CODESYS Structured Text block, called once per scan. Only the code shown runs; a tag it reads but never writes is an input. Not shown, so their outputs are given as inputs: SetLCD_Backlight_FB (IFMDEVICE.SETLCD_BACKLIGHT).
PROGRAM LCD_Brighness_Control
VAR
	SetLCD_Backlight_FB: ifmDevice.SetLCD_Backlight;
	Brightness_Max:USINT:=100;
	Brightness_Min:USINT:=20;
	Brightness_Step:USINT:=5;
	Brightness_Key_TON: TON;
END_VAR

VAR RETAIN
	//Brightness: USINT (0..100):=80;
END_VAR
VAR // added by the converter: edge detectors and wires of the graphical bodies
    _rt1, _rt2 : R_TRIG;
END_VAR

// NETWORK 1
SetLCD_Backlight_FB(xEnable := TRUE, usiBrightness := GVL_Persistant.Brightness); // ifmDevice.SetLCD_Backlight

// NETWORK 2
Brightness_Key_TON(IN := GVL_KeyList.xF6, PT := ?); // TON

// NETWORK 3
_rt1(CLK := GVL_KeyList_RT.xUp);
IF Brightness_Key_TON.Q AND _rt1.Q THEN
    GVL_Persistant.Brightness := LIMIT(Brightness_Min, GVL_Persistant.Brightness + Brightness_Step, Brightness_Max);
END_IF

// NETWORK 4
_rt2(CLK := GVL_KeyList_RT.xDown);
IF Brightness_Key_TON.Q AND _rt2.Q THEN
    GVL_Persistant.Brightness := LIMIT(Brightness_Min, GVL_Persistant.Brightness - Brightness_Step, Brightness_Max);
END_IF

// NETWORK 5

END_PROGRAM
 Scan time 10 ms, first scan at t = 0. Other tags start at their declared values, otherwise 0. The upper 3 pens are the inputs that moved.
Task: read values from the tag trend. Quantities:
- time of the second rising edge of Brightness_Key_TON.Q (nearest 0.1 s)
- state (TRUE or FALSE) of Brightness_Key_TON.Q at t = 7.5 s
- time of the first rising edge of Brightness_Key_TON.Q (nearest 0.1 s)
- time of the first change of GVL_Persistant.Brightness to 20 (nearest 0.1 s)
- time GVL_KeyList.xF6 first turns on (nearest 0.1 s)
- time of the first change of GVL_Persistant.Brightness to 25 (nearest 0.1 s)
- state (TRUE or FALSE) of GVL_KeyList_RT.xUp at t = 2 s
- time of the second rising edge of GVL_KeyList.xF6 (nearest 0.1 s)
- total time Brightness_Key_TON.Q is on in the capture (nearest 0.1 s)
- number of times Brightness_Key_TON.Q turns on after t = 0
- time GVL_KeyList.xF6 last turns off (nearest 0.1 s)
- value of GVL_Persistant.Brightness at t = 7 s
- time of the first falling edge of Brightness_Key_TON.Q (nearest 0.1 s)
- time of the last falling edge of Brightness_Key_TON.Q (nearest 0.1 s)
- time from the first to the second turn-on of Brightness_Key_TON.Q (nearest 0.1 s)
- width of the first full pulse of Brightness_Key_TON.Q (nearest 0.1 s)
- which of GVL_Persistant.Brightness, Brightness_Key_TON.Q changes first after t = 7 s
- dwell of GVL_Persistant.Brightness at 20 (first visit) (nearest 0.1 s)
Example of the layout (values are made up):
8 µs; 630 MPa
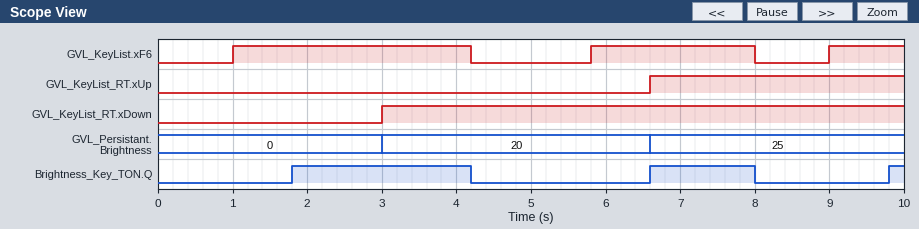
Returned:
6.6 s; TRUE; 1.8 s; 3.0 s; 1.0 s; 6.6 s; FALSE; 5.8 s; 4.0 s; 3; 8.0 s; 25; 4.2 s; 8.0 s; 4.8 s; 2.4 s; Brightness_Key_TON.Q; 3.6 s
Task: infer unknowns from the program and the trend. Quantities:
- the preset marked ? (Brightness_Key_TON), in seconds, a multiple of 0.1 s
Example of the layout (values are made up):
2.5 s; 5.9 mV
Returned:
0.8 s
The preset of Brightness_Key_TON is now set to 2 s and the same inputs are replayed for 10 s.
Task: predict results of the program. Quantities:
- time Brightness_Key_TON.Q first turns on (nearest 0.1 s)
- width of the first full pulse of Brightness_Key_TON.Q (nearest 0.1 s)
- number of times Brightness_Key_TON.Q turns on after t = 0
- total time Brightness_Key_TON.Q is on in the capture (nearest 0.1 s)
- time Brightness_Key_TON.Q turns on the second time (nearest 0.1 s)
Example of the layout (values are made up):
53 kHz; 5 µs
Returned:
3.0 s; 1.2 s; 2; 1.4 s; 7.8 s
